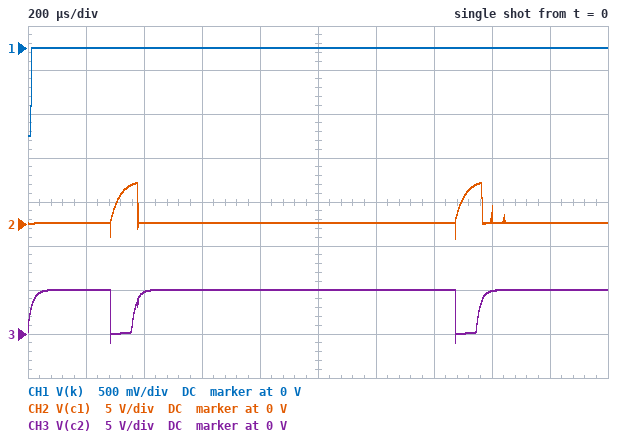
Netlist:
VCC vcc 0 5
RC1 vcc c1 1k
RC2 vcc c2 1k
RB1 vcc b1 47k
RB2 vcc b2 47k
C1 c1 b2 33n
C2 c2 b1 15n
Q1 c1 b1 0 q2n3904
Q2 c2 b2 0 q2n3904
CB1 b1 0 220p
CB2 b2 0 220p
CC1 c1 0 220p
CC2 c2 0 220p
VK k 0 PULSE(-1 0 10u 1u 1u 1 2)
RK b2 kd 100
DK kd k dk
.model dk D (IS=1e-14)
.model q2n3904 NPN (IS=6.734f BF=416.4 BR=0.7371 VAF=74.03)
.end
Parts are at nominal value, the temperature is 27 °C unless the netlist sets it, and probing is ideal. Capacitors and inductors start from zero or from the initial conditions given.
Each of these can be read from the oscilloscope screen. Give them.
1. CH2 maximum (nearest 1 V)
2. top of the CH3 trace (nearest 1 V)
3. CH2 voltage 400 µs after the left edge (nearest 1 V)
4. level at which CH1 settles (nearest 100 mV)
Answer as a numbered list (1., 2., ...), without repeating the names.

1. 5 V
2. 5 V
3. 0 V
4. 0 V
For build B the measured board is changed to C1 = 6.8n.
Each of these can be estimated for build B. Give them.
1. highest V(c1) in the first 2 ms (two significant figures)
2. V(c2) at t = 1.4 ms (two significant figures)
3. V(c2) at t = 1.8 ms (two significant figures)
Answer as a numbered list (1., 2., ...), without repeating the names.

1. 4.8 V
2. 4.9 V
3. 5.0 V
